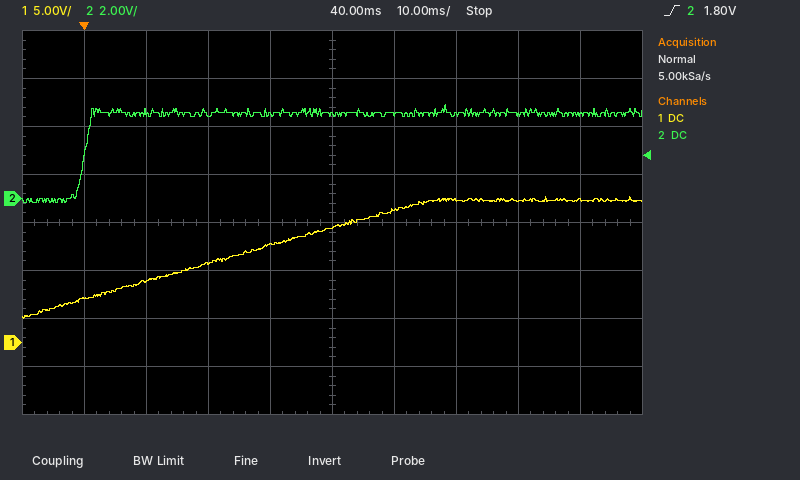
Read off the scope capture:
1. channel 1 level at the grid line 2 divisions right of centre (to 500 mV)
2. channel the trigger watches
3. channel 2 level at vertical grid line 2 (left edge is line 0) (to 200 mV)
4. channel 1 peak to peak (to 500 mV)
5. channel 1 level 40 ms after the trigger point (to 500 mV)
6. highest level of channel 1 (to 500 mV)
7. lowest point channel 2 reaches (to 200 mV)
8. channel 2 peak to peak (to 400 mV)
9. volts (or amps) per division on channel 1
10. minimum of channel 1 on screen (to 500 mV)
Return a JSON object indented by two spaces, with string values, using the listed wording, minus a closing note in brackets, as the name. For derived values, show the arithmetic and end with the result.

{
  "channel 1 level at the grid line 2 divisions right of centre": "15.0 V",
  "channel the trigger watches": "channel 2",
  "channel 2 level at vertical grid line 2 (left edge is line 0)": "3.6 V",
  "channel 1 peak to peak": "15.0 V − (2.5 V) = 12.5 V",
  "channel 1 level 40 ms after the trigger point": "12.0 V",
  "highest level of channel 1": "15.0 V",
  "lowest point channel 2 reaches": "-200 mV",
  "channel 2 peak to peak": "4.0 V",
  "volts (or amps) per division on channel 1": "5 V",
  "minimum of channel 1 on screen": "2.5 V"
}
